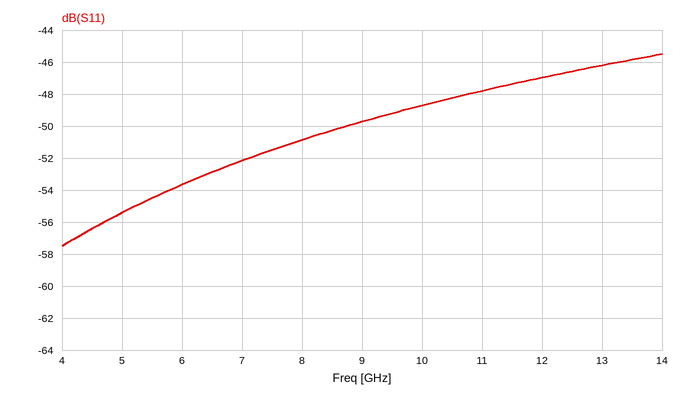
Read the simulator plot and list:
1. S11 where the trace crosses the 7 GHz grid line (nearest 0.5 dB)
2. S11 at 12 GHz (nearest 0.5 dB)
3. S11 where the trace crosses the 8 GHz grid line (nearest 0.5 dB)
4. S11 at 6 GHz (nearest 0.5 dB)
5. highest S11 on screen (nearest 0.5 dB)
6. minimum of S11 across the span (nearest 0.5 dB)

-52.0 dB
-47.0 dB
-51.0 dB
-53.5 dB
-45.5 dB
-57.5 dB
